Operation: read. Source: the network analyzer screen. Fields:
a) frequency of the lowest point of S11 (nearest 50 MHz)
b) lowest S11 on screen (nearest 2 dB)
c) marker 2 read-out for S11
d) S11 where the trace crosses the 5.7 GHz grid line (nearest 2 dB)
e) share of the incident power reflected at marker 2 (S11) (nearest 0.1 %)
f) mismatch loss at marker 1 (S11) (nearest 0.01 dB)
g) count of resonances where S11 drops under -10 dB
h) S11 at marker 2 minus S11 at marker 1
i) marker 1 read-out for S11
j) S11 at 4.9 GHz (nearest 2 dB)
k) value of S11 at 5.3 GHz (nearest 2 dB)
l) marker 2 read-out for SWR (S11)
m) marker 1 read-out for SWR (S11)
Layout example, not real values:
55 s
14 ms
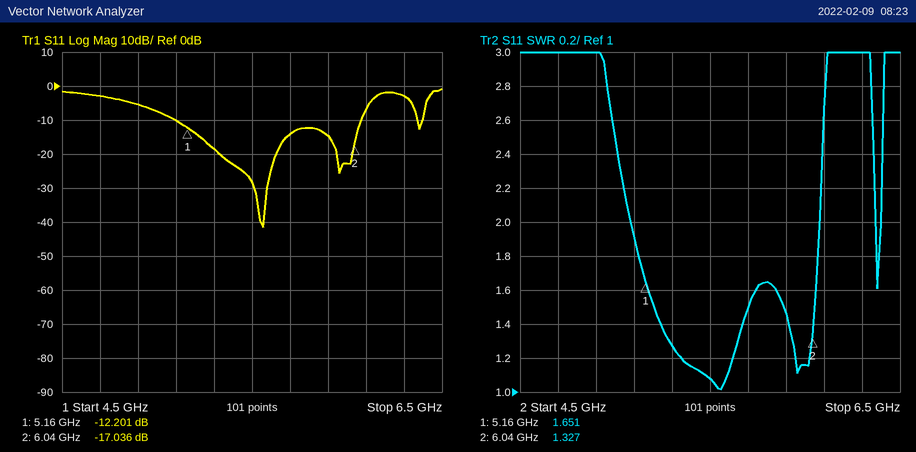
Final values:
5.55 GHz
-42 dB
-17.036 dB
-14 dB
2.0 %
0.27 dB
3
-4.835 dB
-12.201 dB
-6 dB
-18 dB
1.327
1.651
